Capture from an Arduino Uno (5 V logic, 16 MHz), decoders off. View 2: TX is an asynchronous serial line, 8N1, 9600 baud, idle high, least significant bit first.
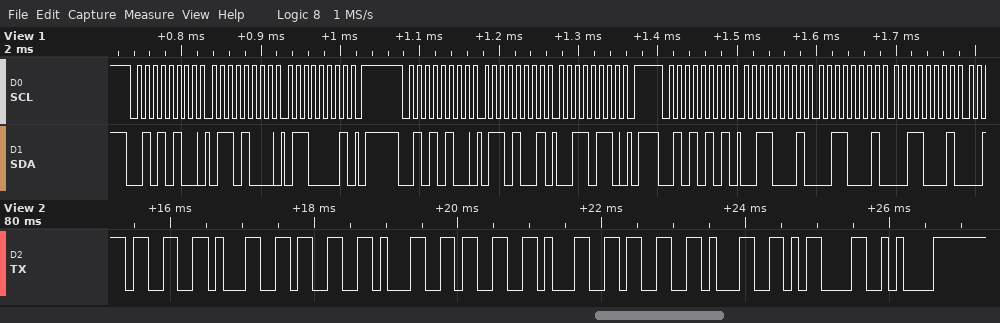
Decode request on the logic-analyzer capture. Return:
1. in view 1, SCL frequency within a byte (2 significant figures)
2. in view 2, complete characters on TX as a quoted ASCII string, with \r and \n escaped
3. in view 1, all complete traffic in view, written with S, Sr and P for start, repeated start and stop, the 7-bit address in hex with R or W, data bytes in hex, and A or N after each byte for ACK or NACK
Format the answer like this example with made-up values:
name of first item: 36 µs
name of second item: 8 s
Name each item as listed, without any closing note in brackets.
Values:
in view 1, SCL frequency within a byte: 100 kHz
in view 2, complete characters on TX as a quoted ASCII string, with \r and \n escaped: "31313131\r\n"
in view 1, all complete traffic in view, written with S, Sr and P for start, repeated start and stop, the 7-bit address in hex with R or W, data bytes in hex, and A or N after each byte for ACK or NACK: S 2AW A 68 A 61 A P S 2AW A 69 A 36 A P S 2AR A 31 A 31 A 31 A
